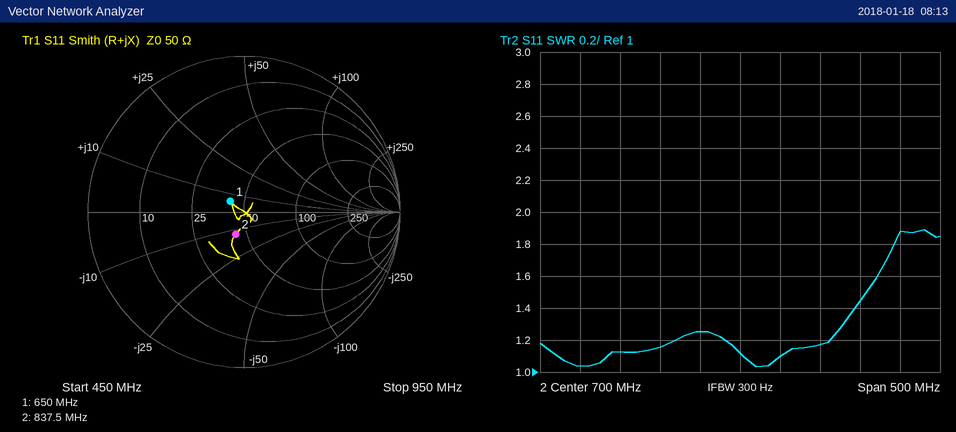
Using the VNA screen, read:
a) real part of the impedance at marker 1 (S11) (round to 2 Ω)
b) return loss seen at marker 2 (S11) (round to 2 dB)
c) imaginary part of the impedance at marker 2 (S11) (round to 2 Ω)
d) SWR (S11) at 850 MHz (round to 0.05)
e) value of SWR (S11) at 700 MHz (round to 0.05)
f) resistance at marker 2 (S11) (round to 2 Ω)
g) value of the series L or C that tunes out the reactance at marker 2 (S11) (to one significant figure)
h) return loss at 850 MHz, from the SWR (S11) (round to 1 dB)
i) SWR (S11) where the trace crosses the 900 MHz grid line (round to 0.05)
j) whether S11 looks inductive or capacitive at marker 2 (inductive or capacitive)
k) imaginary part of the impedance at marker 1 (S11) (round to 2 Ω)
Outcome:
42 Ω
16 dB
-12 Ω
1.45
1.10
44 Ω
2 nH
15 dB
1.90
capacitive
+6 Ω
